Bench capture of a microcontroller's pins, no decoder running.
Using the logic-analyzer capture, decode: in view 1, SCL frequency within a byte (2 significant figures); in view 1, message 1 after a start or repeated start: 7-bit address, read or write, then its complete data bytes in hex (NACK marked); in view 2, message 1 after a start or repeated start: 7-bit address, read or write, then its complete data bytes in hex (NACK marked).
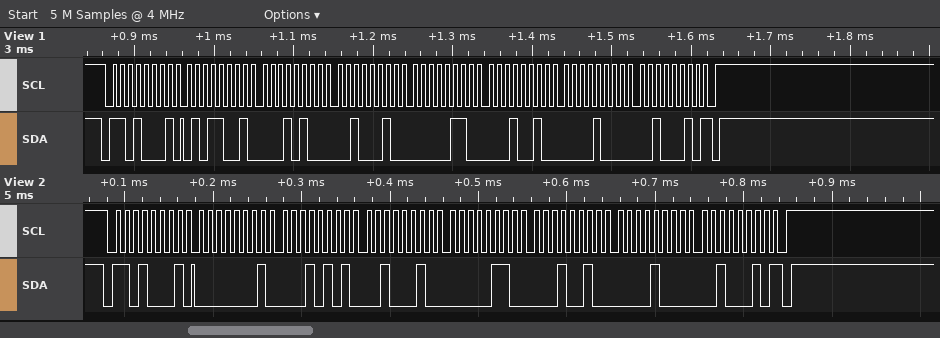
100 kHz
0x68 read: 59 14 22 06 12 08 22 NACK
0x68 read: 01 15 22 06 12 08 22 NACK
